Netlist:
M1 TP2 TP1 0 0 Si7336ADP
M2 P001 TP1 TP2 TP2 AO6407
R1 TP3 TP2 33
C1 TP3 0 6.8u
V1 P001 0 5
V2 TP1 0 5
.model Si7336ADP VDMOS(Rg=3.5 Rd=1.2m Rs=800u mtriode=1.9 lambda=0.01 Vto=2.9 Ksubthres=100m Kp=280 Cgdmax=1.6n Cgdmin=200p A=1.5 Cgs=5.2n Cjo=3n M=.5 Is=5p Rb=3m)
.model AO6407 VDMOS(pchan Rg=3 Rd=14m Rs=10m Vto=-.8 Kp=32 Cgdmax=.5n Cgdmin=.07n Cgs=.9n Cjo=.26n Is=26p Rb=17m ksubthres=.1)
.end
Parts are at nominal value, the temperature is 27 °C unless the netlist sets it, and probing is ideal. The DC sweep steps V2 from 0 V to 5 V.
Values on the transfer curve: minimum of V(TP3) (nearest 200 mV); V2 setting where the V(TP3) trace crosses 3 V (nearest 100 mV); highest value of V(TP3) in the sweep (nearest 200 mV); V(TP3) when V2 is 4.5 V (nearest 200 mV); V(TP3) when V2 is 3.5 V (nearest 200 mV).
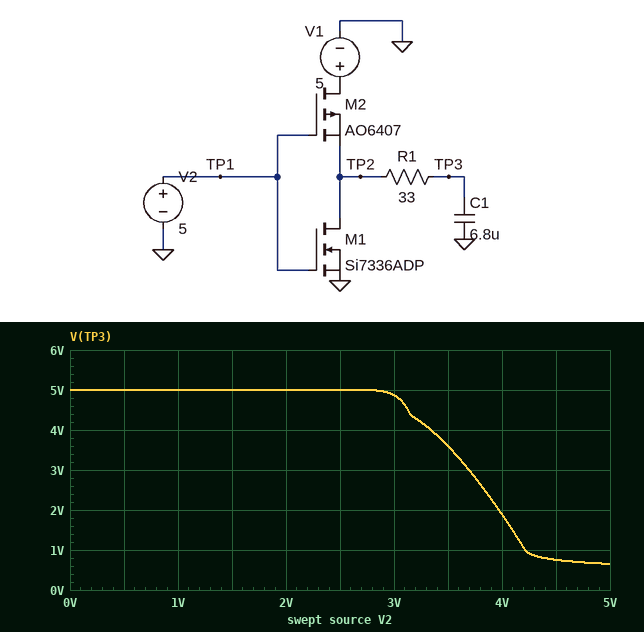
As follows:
600 mV
3.7 V
5.0 V
800 mV
3.6 V
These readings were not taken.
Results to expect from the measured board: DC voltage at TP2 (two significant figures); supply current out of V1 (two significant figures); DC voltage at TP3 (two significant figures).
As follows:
650 mV
210 A
650 mV
